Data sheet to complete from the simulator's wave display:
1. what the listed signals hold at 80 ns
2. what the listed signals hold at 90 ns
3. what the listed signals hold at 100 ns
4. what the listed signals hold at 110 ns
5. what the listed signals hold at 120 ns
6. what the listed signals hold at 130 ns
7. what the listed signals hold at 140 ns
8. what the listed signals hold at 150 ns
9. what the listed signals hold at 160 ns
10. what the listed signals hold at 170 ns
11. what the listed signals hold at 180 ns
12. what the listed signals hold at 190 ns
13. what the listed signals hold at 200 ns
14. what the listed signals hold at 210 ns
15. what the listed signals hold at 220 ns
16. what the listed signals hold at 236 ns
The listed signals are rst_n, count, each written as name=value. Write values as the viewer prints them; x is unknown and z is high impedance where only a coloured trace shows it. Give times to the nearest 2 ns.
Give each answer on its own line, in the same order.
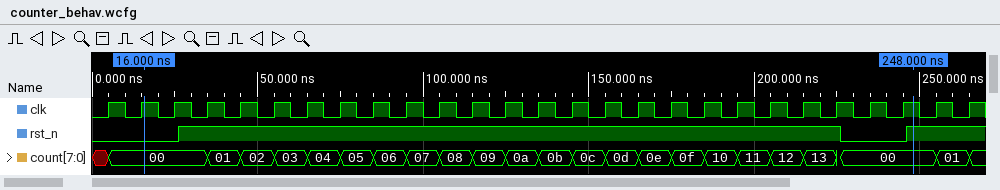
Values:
rst_n=1, count=05
rst_n=1, count=06
rst_n=1, count=07
rst_n=1, count=08
rst_n=1, count=09
rst_n=1, count=0a
rst_n=1, count=0b
rst_n=1, count=0c
rst_n=1, count=0d
rst_n=1, count=0e
rst_n=1, count=0f
rst_n=1, count=10
rst_n=1, count=11
rst_n=1, count=12
rst_n=1, count=13
rst_n=0, count=00
